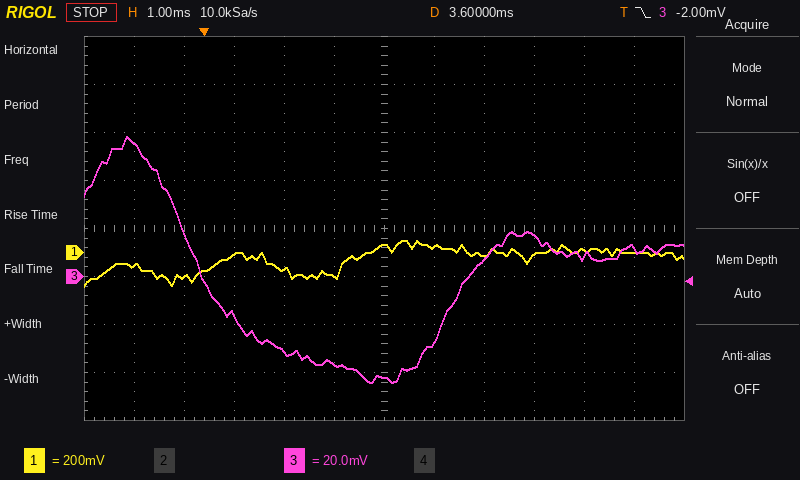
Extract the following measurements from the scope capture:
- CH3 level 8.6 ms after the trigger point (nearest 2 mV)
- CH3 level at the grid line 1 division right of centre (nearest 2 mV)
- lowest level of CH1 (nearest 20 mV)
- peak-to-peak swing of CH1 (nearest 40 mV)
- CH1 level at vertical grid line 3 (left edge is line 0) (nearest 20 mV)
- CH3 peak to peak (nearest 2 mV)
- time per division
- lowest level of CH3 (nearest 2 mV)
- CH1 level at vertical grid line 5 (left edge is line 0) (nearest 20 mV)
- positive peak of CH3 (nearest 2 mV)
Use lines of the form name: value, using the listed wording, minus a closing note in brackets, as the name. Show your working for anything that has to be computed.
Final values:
CH3 level 8.6 ms after the trigger point: 12 mV
CH3 level at the grid line 1 division right of centre: -28 mV
lowest level of CH1: -140 mV
peak-to-peak swing of CH1: 200 mV
CH1 level at vertical grid line 3 (left edge is line 0): 0 mV
CH3 peak to peak: 58 mV − (-44 mV) = 102 mV
time per division: 1 ms
lowest level of CH3: -44 mV
CH1 level at vertical grid line 5 (left edge is line 0): -100 mV
positive peak of CH3: 58 mV
